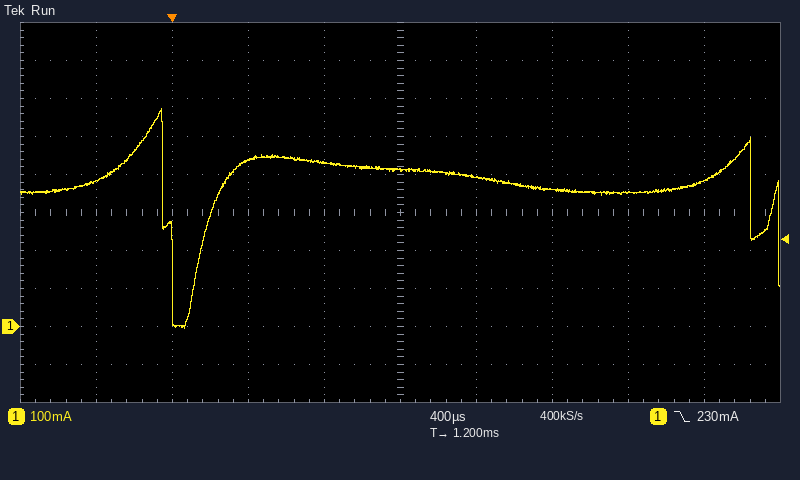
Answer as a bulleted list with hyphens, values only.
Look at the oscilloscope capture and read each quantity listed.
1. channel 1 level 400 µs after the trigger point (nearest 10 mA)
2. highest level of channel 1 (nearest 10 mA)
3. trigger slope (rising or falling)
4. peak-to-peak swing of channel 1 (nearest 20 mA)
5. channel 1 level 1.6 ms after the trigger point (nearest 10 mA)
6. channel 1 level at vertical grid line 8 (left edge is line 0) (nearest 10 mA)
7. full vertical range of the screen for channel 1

- 440 mA
- 570 mA
- falling
- 580 mA
- 390 mA
- 350 mA
- 1 A
